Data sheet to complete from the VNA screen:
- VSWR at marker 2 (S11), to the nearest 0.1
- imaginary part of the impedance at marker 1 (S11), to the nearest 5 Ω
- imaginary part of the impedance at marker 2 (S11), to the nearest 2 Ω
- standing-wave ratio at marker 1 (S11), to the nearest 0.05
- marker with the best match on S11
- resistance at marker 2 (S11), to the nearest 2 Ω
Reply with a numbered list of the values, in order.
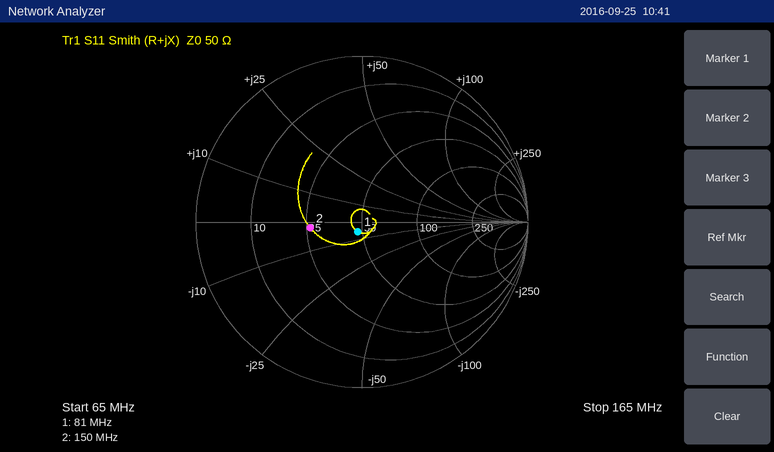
1. 1.9
2. -5 Ω
3. -2 Ω
4. 1.15
5. marker 1
6. 26 Ω
